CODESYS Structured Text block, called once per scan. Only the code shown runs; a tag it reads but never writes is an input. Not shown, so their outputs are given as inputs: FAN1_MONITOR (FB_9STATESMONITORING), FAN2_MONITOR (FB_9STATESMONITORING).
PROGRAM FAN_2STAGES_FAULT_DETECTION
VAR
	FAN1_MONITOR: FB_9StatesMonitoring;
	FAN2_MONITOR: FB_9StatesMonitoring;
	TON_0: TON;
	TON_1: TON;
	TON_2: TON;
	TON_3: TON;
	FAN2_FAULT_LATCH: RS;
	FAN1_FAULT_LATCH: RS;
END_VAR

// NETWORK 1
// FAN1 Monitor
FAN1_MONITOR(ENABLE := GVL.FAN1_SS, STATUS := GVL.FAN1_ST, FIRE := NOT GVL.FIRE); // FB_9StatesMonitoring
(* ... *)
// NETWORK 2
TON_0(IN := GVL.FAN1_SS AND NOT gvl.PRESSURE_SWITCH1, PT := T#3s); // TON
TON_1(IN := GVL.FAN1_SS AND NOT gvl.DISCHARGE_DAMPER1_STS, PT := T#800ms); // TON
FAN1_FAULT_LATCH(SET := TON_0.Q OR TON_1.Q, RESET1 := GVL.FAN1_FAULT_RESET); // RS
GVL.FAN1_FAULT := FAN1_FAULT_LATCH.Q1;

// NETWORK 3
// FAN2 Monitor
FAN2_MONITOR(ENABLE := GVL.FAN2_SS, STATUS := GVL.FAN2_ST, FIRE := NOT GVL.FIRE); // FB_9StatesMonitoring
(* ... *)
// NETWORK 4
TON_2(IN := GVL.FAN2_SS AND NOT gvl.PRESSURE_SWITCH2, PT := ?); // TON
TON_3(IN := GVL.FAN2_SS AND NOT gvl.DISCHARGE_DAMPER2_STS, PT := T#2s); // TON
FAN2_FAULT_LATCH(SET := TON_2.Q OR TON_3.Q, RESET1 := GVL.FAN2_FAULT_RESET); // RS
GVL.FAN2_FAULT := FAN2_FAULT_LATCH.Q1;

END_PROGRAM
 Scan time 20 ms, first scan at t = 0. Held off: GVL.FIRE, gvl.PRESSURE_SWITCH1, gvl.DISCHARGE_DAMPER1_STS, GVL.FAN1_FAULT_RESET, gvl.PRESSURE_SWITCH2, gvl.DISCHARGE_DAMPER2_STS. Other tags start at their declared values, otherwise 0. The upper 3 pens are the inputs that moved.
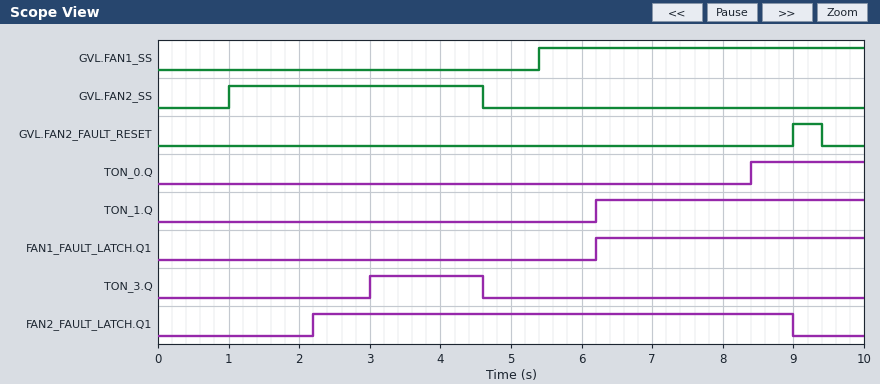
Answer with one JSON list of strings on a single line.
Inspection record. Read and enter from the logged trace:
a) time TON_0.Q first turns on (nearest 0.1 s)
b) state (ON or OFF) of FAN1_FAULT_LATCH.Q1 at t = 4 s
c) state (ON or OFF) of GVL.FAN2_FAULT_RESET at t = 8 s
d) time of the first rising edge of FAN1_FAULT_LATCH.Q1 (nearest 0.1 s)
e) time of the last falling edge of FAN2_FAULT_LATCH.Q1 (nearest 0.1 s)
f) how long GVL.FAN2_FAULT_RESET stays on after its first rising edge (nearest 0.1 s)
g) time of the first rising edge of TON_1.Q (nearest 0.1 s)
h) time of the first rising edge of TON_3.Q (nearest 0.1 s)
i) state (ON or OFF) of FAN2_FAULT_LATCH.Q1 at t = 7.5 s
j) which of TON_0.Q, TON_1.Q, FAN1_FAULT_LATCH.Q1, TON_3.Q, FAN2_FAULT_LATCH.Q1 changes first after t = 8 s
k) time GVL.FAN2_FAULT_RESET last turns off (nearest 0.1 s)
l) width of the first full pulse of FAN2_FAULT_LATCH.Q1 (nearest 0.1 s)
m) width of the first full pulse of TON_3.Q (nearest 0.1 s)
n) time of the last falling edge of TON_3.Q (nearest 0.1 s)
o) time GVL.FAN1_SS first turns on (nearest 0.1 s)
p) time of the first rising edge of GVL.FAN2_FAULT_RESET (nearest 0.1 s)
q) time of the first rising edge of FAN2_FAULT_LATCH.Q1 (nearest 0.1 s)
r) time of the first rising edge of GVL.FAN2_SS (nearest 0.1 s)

["8.4 s", "OFF", "OFF", "6.2 s", "9.0 s", "0.4 s", "6.2 s", "3.0 s", "ON", "TON_0.Q", "9.4 s", "6.8 s", "1.6 s", "4.6 s", "5.4 s", "9.0 s", "2.2 s", "1.0 s"]
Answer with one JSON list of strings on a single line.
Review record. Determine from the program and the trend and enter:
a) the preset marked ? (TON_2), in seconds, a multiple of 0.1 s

["1.2 s"]
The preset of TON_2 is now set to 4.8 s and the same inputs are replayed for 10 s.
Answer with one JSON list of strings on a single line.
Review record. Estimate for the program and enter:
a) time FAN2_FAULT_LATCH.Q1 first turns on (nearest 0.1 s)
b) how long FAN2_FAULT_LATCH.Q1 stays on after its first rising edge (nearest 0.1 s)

["3.0 s", "6.0 s"]
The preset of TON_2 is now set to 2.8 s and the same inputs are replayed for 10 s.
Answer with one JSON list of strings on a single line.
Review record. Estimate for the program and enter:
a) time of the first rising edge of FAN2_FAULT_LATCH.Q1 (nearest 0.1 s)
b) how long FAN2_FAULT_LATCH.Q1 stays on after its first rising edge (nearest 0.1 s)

["3.0 s", "6.0 s"]
